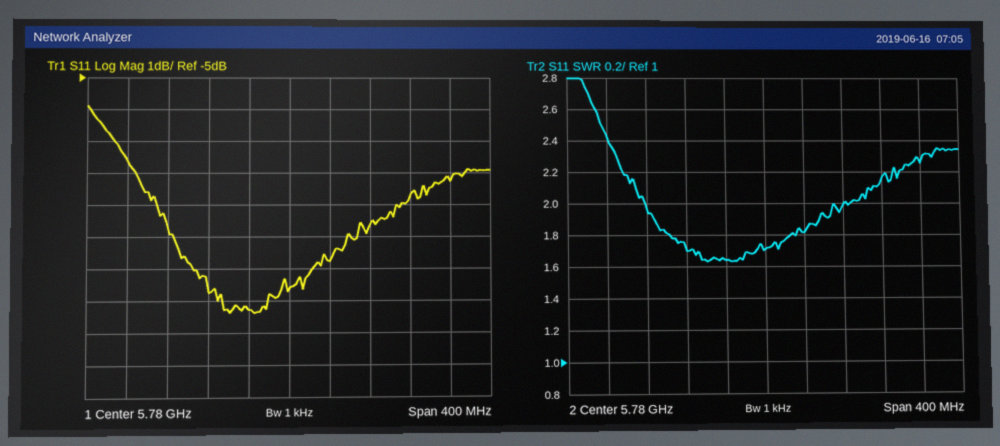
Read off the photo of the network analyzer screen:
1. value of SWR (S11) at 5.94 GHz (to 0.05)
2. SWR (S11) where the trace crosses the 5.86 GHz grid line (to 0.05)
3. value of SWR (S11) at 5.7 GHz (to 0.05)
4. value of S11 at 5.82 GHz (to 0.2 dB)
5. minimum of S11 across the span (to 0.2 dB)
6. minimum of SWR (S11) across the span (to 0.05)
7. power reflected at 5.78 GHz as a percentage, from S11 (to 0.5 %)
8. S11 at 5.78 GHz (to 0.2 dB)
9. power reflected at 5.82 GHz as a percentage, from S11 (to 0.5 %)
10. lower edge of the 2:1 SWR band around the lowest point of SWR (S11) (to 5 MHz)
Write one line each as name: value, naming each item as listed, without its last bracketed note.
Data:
value of SWR (S11) at 5.94 GHz: 2.25
SWR (S11) where the trace crosses the 5.86 GHz grid line: 2.00
value of SWR (S11) at 5.7 GHz: 1.70
value of S11 at 5.82 GHz: -10.8 dB
minimum of S11 across the span: -12.4 dB
minimum of SWR (S11) across the span: 1.65
power reflected at 5.78 GHz as a percentage, from S11: 7.0 %
S11 at 5.78 GHz: -11.6 dB
power reflected at 5.82 GHz as a percentage, from S11: 8.5 %
lower edge of the 2:1 SWR band around the lowest point of SWR (S11): 5.660 GHz
